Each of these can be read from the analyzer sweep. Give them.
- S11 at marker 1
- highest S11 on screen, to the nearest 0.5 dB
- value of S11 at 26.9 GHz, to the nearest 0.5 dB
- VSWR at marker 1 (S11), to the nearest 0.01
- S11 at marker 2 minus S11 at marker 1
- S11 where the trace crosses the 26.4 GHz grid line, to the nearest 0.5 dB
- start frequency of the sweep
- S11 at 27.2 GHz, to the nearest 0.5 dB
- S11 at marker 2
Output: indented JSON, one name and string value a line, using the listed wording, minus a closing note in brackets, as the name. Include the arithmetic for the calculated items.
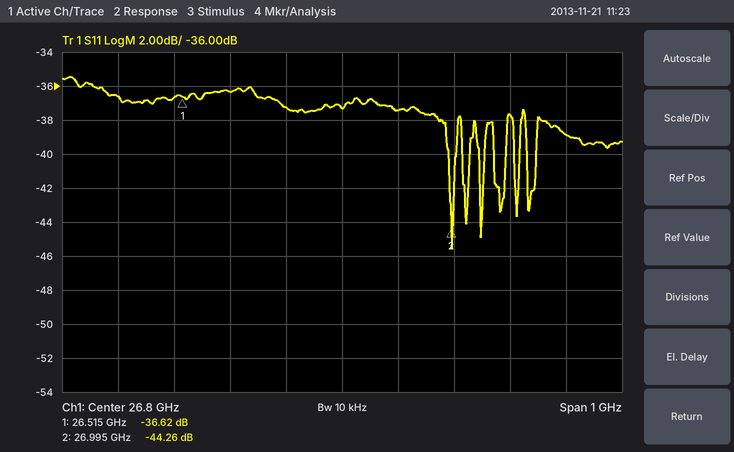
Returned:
{
  "S11 at marker 1": "-36.62 dB",
  "highest S11 on screen, to the nearest 0.5 dB": "-35.5 dB",
  "value of S11 at 26.9 GHz, to the nearest 0.5 dB": "-37.5 dB",
  "VSWR at marker 1 (S11), to the nearest 0.01": "(1 + 0.0148)/(1 − 0.0148) ≈ 1.03",
  "S11 at marker 2 minus S11 at marker 1": "-44.26 − (-36.62) = -7.64 dB",
  "S11 where the trace crosses the 26.4 GHz grid line, to the nearest 0.5 dB": "-36.5 dB",
  "start frequency of the sweep": "26.3 GHz",
  "S11 at 27.2 GHz, to the nearest 0.5 dB": "-39.0 dB",
  "S11 at marker 2": "-44.26 dB"
}
